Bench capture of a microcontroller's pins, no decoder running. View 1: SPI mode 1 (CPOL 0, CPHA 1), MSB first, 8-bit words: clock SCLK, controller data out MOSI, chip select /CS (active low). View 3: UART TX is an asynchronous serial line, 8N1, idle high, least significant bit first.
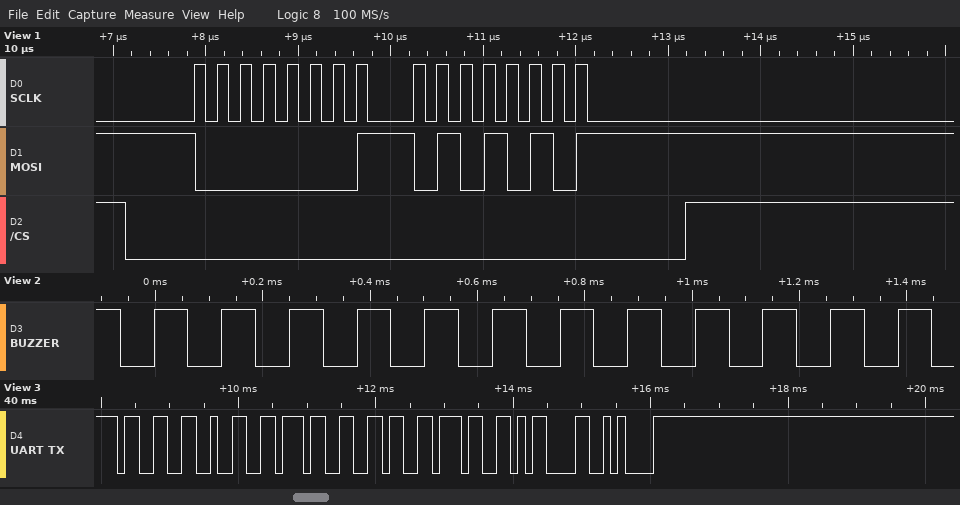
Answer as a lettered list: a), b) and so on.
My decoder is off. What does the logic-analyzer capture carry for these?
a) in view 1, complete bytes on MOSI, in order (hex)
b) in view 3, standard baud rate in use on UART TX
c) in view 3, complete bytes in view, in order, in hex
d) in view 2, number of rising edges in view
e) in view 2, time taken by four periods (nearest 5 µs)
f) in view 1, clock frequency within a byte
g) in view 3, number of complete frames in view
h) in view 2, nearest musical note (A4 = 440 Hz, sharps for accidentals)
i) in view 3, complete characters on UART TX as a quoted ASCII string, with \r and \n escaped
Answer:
a) 01 55
b) 9600 baud
c) 0x33 0x32 0x37 0x36 0x37 0x0D 0x0A
d) 12
e) 505 µs
f) 4 MHz
g) 7
h) B8
i) "32767\r\n"
